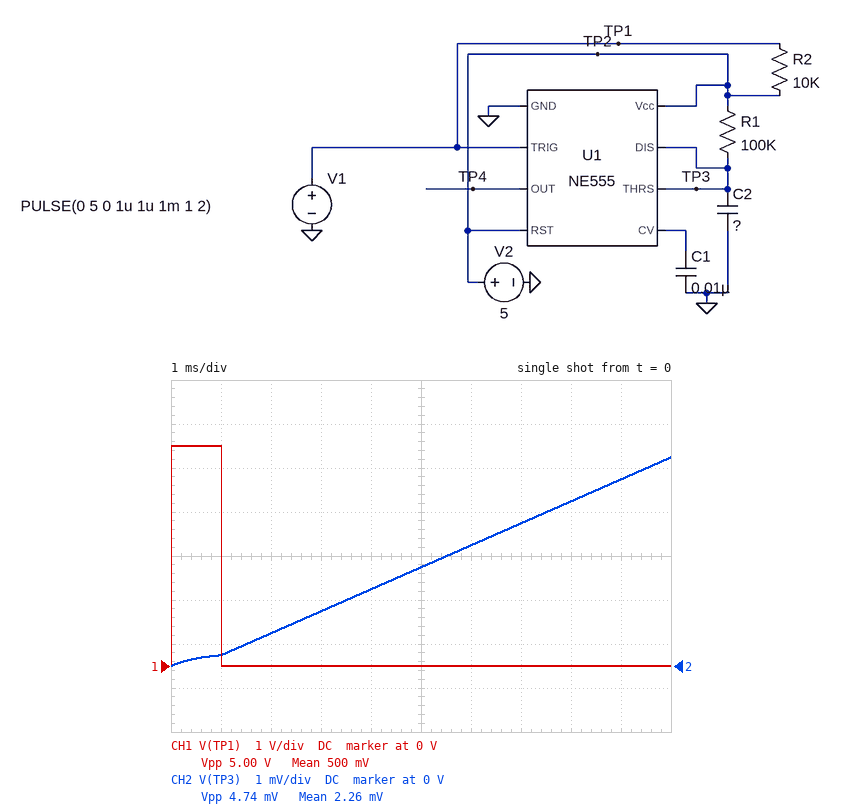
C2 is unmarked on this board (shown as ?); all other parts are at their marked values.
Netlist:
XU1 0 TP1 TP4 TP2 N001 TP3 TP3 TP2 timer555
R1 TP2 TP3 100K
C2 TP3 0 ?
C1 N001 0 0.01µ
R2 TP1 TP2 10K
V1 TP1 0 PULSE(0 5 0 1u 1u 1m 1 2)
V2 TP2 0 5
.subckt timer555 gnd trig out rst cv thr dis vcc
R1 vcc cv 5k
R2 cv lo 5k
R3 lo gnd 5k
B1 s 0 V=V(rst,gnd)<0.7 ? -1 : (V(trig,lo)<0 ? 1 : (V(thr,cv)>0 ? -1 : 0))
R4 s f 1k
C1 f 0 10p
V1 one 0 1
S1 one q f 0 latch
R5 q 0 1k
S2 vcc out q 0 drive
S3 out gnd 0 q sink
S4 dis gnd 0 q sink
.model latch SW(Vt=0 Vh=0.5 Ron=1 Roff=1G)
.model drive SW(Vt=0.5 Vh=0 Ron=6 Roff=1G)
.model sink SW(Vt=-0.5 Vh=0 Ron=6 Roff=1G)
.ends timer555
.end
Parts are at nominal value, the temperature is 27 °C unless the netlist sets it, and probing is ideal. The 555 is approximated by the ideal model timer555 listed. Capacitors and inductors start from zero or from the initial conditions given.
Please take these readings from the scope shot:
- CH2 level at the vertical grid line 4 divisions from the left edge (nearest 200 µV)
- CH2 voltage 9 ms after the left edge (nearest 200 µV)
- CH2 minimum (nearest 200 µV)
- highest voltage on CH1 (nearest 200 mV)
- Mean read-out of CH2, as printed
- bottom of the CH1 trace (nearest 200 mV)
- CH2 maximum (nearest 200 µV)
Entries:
1.8 mV
4.2 mV
0 V
5.0 V
2.26 mV
0 V
4.8 mV
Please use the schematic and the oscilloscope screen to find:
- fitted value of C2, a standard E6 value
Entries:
100 µF
